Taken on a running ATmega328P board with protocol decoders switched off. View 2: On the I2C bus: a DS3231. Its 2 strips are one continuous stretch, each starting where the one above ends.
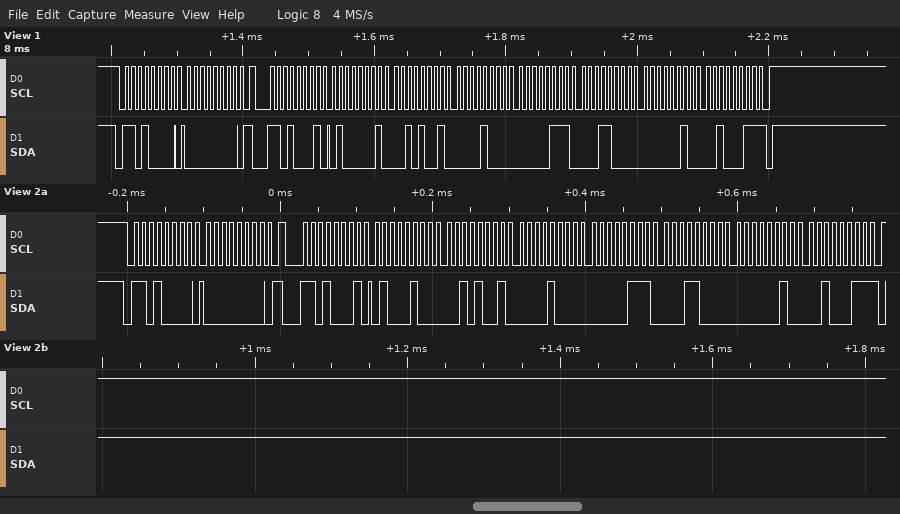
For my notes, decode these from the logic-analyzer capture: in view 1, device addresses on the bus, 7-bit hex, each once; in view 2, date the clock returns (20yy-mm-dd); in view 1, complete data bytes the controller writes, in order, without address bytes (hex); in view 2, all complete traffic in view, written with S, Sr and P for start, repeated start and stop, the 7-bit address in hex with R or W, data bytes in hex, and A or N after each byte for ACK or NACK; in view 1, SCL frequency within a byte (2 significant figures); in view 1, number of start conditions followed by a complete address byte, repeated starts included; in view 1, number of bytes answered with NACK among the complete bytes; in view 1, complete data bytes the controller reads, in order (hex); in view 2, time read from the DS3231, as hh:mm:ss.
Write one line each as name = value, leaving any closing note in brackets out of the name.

in view 1, device addresses on the bus, 7-bit hex, each once = 0x68
in view 2, date the clock returns = 2023-02-18
in view 1, complete data bytes the controller writes, in order, without address bytes = 00
in view 2, all complete traffic in view, written with S, Sr and P for start, repeated start and stop, the 7-bit address in hex with R or W, data bytes in hex, and A or N after each byte for ACK or NACK = S 68W A 00 A Sr 68R A 44 A 29 A 08 A 07 A 18 A 02 A 23 N P
in view 1, SCL frequency within a byte = 100 kHz
in view 1, number of start conditions followed by a complete address byte, repeated starts included = 2
in view 1, number of bytes answered with NACK among the complete bytes = 1
in view 1, complete data bytes the controller reads, in order = 41 29 08 07 18 02 23
in view 2, time read from the DS3231, as hh:mm:ss = 08:29:44
